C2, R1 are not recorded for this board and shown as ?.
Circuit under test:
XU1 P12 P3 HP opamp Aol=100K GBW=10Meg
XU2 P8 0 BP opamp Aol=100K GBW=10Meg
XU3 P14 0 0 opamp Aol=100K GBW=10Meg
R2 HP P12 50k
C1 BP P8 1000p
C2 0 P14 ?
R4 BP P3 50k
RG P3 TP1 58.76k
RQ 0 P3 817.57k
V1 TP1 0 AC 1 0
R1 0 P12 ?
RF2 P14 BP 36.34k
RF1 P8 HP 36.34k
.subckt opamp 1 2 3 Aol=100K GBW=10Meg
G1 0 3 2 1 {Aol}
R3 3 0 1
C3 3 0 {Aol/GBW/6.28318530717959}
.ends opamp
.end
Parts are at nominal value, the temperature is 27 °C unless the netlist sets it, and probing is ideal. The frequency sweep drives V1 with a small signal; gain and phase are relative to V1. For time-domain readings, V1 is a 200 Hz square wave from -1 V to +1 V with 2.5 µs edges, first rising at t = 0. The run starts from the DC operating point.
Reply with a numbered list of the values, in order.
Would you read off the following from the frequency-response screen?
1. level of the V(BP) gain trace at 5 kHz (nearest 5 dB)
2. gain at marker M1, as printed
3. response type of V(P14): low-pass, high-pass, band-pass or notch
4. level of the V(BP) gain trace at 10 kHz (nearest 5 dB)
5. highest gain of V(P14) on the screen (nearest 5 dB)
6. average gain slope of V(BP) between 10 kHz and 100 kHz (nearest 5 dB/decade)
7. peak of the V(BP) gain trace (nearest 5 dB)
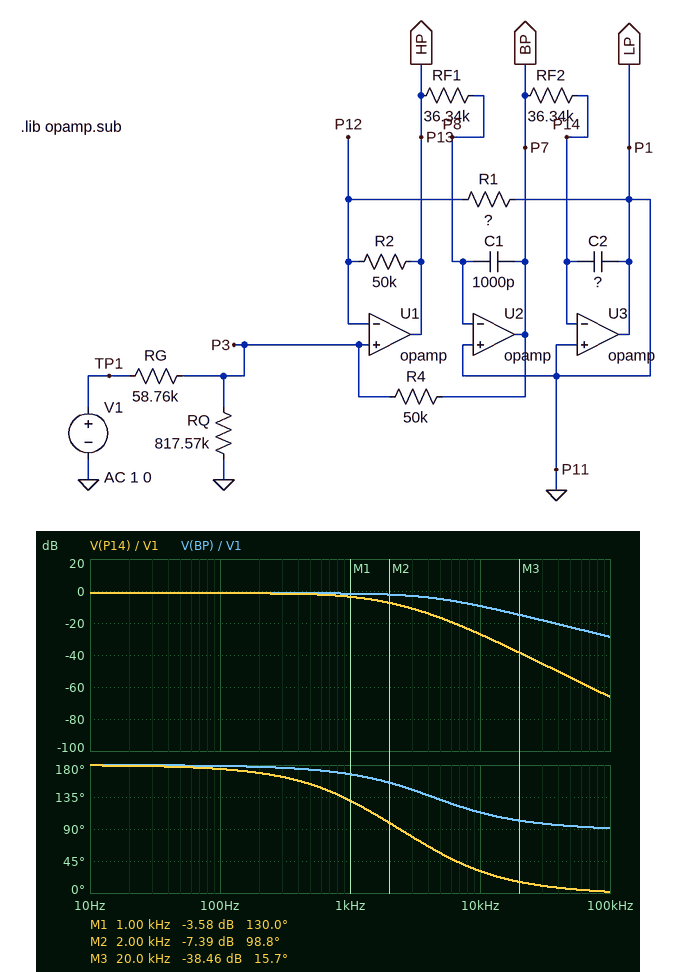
1. -5 dB
2. -3.58 dB
3. low-pass
4. -10 dB
5. 0 dB
6. -20 dB/decade
7. 0 dB
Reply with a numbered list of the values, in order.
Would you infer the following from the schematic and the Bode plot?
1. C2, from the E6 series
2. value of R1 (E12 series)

1. 3.3 nF
2. 56 kΩ
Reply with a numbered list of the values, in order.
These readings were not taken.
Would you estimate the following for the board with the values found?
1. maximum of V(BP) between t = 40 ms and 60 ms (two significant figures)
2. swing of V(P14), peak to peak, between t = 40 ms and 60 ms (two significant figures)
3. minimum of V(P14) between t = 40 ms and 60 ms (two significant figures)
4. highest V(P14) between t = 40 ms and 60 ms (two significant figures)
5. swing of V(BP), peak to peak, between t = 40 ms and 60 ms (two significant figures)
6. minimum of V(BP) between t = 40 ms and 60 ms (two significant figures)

1. 850 mV
2. 1.7 V
3. -850 mV
4. 850 mV
5. 1.7 V
6. -850 mV
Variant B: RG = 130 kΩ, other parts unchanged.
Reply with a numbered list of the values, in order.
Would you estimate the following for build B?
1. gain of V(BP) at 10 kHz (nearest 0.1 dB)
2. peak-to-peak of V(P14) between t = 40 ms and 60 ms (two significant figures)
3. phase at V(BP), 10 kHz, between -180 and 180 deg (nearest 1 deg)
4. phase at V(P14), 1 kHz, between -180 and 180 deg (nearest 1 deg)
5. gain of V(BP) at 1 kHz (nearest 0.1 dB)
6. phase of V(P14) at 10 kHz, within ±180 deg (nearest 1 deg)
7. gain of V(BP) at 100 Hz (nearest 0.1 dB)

1. -14.4 dB
2. 770 mV
3. 120 deg
4. 133 deg
5. -8.4 dB
6. 37 deg
7. -8.3 dB
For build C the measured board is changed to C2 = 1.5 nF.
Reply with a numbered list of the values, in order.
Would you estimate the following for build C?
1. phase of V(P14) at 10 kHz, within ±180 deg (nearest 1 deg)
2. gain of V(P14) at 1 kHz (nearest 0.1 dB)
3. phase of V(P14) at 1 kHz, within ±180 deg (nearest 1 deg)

1. 40 deg
2. -2.1 dB
3. 148 deg
